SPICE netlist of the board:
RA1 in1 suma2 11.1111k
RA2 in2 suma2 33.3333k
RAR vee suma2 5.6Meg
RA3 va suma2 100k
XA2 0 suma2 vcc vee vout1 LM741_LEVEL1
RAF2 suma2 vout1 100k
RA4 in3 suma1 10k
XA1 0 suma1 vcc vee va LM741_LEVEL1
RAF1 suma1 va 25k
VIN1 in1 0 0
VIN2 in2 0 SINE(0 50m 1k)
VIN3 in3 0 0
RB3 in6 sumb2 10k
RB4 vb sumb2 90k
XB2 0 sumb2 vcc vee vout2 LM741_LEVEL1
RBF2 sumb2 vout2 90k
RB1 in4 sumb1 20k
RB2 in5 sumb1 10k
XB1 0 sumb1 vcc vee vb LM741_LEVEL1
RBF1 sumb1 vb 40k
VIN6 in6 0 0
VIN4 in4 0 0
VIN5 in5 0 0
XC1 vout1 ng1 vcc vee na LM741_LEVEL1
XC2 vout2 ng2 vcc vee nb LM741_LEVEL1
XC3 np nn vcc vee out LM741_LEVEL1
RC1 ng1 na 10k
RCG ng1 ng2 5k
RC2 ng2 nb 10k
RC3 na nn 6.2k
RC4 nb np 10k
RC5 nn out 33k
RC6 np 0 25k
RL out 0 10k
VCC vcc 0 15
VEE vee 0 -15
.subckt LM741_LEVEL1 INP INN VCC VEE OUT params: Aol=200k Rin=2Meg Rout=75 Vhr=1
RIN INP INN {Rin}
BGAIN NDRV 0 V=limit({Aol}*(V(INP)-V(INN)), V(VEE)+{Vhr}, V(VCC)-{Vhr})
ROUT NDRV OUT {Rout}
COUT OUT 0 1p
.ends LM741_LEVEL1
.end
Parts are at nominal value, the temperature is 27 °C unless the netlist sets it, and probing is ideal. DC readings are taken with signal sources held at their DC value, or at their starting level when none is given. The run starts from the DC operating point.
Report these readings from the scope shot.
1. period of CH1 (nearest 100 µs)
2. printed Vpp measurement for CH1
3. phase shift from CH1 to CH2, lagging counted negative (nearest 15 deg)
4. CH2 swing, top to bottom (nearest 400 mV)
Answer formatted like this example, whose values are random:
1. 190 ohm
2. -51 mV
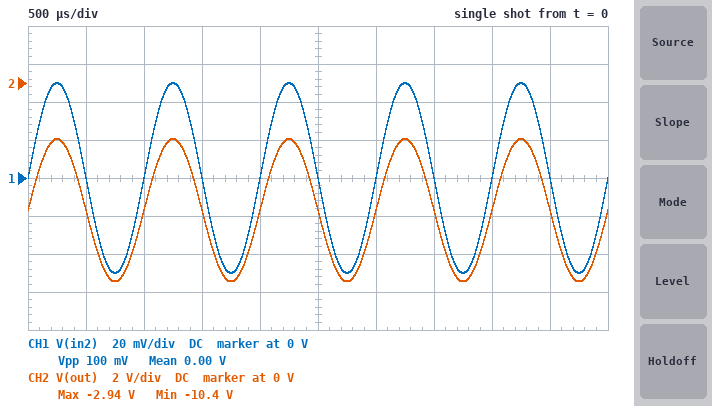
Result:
1. 1.0 ms
2. 100 mV
3. 0 deg
4. 7.6 V
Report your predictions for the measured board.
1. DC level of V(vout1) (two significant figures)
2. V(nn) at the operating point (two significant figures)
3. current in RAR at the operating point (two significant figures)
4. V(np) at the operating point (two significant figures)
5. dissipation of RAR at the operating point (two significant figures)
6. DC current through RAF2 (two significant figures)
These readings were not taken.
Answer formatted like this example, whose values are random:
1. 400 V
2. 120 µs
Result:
1. 270 mV
2. -380 mV
3. 2.7 µA
4. -380 mV
5. 40 µW
6. 2.7 µA
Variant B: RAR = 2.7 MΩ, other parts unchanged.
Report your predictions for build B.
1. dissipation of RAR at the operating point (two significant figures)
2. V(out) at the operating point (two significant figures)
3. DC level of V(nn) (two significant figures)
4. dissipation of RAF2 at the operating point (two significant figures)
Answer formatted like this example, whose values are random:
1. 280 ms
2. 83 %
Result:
1. 83 µW
2. -14 V
3. -790 mV
4. 3.1 µW
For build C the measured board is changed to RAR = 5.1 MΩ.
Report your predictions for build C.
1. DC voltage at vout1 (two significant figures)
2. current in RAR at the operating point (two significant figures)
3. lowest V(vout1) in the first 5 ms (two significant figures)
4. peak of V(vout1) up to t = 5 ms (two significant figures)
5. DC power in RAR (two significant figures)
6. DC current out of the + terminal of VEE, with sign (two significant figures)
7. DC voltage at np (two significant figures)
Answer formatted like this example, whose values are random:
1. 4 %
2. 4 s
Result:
1. 290 mV
2. 2.9 µA
3. 140 mV
4. 440 mV
5. 44 µW
6. -2.9 µA
7. -420 mV
